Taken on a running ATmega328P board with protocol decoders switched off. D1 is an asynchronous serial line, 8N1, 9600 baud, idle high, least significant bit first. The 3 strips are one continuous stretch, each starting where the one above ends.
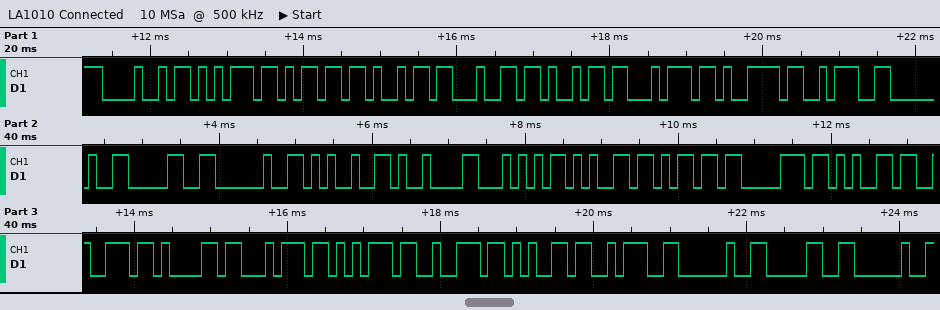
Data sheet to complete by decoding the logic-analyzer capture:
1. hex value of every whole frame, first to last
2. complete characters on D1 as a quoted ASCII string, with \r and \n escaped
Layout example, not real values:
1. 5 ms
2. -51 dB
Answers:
1. 48 75 6D 69 64 69 74 79 3A 20 30 20 25 09 54 65 6D 70 65 72 61 74 75 72 65 3A 20 30 20
2. "Humidity: 0 %\tTemperature: 0 "
